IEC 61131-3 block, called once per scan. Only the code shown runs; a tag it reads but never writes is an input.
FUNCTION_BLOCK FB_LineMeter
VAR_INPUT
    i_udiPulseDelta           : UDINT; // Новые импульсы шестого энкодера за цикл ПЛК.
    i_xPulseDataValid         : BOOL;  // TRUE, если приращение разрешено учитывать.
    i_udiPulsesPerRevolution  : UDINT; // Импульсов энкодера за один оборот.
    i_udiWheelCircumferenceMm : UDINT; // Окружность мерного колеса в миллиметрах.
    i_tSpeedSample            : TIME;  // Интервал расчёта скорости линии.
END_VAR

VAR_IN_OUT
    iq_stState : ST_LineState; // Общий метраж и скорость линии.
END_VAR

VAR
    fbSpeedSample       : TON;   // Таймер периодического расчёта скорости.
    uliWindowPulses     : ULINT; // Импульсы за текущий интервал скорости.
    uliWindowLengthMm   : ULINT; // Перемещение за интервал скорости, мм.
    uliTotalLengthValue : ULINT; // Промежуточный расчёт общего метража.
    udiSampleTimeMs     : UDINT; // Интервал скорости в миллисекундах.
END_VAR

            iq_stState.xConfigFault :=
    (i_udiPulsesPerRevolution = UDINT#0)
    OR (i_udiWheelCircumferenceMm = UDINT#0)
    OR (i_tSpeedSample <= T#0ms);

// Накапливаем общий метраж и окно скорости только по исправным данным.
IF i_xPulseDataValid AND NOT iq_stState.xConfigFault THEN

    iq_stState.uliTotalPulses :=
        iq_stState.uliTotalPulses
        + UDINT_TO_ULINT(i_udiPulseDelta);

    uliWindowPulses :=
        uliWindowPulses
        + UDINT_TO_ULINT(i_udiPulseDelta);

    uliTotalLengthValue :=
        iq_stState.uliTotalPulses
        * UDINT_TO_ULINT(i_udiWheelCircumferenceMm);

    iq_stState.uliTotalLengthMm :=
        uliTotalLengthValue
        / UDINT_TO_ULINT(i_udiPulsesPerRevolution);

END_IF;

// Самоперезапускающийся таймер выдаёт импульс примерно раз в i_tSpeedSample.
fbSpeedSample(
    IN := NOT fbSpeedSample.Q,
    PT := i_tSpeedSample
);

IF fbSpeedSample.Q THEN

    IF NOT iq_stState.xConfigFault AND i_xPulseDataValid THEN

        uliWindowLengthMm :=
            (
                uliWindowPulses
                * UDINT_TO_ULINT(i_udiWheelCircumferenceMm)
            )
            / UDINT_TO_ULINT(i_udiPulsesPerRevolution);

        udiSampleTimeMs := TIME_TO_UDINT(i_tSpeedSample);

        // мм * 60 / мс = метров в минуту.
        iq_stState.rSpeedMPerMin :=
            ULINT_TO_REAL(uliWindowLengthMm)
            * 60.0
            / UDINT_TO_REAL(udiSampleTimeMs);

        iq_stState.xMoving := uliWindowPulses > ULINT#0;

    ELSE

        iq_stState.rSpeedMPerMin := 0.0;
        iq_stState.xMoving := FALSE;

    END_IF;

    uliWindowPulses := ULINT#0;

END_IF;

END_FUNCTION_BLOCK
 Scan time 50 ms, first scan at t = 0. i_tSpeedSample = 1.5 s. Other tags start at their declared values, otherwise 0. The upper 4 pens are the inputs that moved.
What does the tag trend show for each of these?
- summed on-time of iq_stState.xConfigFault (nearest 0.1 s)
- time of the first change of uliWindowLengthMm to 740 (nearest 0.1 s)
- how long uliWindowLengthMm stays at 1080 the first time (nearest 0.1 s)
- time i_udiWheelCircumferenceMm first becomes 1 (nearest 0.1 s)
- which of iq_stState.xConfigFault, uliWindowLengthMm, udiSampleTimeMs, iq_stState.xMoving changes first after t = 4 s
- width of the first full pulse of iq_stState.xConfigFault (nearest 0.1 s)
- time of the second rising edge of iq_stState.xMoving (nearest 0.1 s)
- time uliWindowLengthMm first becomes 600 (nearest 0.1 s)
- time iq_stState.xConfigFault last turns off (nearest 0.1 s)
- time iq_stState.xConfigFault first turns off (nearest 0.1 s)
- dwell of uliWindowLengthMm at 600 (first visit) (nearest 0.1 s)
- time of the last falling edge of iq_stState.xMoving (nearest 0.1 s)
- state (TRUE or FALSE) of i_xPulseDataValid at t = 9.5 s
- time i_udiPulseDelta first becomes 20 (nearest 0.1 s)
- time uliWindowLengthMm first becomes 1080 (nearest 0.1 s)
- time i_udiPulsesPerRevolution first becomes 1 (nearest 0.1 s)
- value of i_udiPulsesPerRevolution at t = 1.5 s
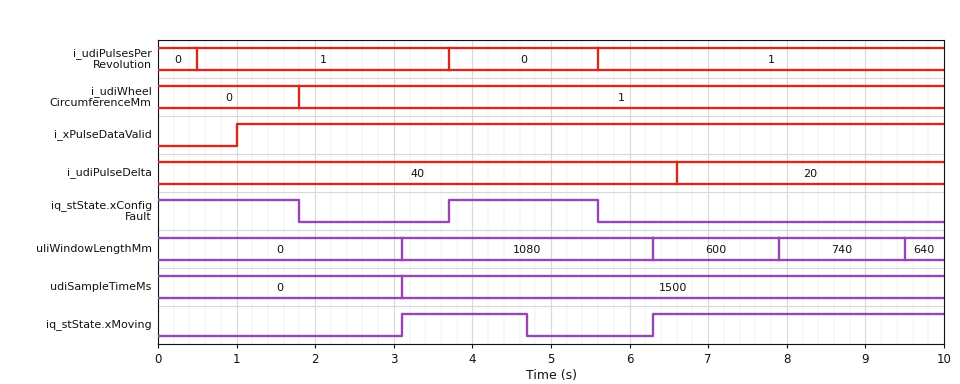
3.7 s
7.9 s
3.2 s
1.8 s
iq_stState.xMoving
1.9 s
6.3 s
6.3 s
5.6 s
1.8 s
1.6 s
4.7 s
TRUE
6.6 s
3.1 s
0.5 s
1
